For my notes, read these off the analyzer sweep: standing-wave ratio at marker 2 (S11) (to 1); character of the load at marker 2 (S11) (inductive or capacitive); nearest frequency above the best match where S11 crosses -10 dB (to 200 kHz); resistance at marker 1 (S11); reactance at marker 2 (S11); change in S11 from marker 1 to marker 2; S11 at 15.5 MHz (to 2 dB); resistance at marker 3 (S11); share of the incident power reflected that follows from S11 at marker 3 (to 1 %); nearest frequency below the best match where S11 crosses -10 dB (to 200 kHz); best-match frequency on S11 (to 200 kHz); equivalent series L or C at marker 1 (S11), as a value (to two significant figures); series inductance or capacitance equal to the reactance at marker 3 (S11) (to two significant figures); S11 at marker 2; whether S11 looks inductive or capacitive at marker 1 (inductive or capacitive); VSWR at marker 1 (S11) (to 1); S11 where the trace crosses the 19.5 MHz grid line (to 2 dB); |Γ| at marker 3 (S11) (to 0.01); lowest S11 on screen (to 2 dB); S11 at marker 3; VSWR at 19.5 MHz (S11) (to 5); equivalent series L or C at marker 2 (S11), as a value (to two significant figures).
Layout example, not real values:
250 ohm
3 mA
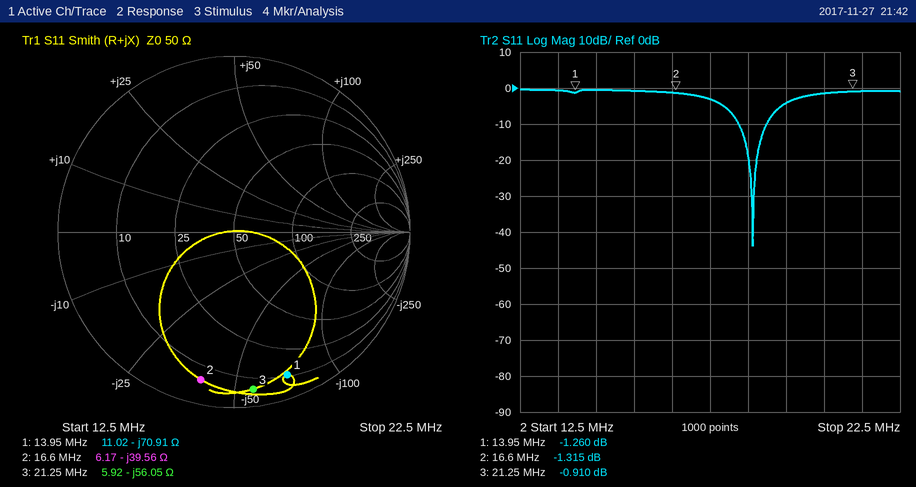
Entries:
13
capacitive
19.0 MHz
11.02 Ω
-39.56 Ω
-0.055 dB
0 dB
5.92 Ω
81 %
18.2 MHz
18.6 MHz
160 pF
130 pF
-1.315 dB
capacitive
14
-4 dB
0.90
-44 dB
-0.910 dB
5
240 pF
